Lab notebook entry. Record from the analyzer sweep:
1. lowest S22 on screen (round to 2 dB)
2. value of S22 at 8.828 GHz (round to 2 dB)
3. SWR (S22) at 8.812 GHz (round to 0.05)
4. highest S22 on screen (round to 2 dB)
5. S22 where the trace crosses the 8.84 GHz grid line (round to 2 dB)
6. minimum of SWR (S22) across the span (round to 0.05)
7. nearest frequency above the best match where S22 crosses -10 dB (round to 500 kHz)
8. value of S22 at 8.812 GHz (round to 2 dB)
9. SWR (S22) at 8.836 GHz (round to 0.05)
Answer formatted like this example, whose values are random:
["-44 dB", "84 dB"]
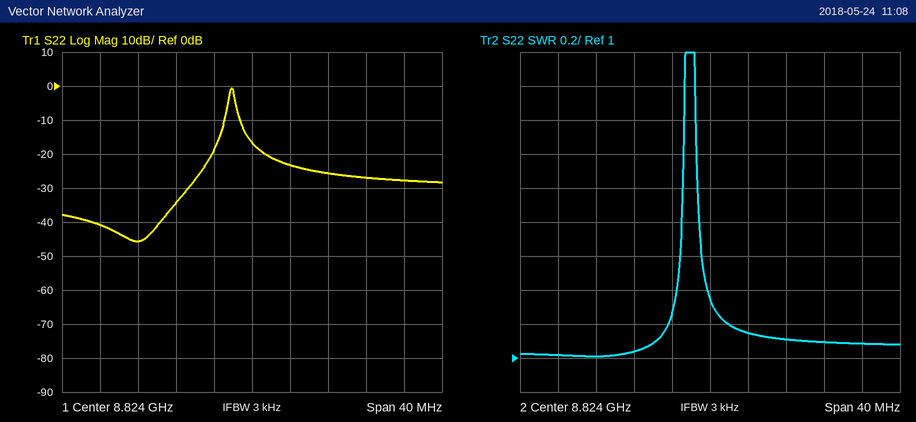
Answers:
["-46 dB", "-24 dB", "1.00", "0 dB", "-28 dB", "1.00", "8.8210 GHz", "-46 dB", "1.10"]
